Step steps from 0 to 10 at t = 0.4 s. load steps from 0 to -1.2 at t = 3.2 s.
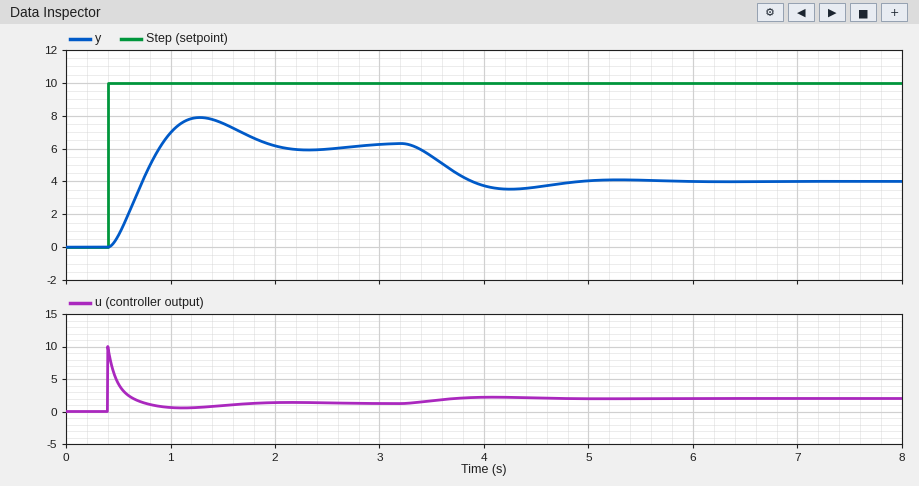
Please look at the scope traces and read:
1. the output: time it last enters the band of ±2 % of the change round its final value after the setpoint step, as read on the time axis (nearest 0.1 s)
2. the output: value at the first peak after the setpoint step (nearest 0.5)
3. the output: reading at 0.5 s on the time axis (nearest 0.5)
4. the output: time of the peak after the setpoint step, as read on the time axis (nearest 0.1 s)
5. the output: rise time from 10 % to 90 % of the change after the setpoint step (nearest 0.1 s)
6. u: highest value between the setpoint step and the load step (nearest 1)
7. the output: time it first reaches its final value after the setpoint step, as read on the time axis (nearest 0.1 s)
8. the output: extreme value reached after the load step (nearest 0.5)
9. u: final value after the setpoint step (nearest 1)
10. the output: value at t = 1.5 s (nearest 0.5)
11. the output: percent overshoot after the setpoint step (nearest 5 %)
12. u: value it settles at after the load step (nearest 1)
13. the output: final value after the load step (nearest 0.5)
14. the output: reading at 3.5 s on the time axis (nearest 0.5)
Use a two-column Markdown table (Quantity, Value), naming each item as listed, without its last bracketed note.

| Quantity | Value |
|---|---|
| the output: time it last enters the band of ±2 % of the change round its final value after the setpoint step, as read on the time axis | 2.8 s |
| the output: value at the first peak after the setpoint step | 8.0 |
| the output: reading at 0.5 s on the time axis | 0.5 |
| the output: time of the peak after the setpoint step, as read on the time axis | 1.3 s |
| the output: rise time from 10 % to 90 % of the change after the setpoint step | 0.4 s |
| u: highest value between the setpoint step and the load step | 10 |
| the output: time it first reaches its final value after the setpoint step, as read on the time axis | 0.9 s |
| the output: extreme value reached after the load step | 3.5 |
| u: final value after the setpoint step | 1 |
| the output: value at t = 1.5 s | 7.5 |
| the output: percent overshoot after the setpoint step | 25 % |
| u: value it settles at after the load step | 2 |
| the output: final value after the load step | 4.0 |
| the output: reading at 3.5 s on the time axis | 5.5 |
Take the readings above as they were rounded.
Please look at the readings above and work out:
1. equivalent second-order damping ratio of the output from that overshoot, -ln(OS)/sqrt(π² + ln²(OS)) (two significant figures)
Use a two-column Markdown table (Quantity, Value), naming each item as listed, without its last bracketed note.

| Quantity | Value |
|---|---|
| equivalent second-order damping ratio of the output from that overshoot, -ln(OS)/sqrt(π² + ln²(OS)) | 0.40 |
